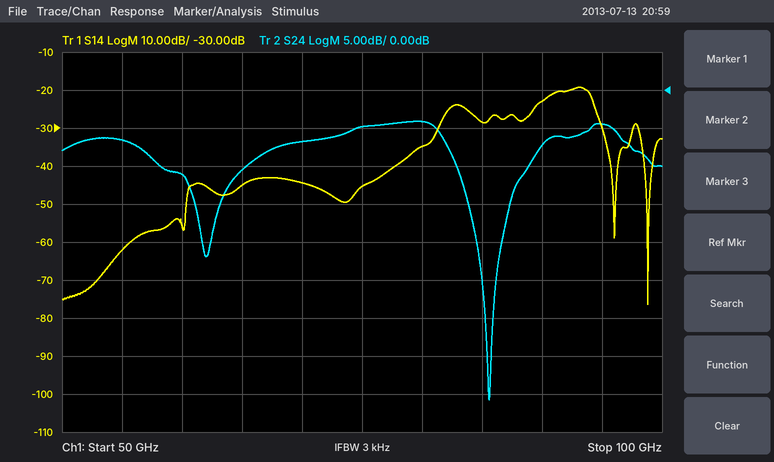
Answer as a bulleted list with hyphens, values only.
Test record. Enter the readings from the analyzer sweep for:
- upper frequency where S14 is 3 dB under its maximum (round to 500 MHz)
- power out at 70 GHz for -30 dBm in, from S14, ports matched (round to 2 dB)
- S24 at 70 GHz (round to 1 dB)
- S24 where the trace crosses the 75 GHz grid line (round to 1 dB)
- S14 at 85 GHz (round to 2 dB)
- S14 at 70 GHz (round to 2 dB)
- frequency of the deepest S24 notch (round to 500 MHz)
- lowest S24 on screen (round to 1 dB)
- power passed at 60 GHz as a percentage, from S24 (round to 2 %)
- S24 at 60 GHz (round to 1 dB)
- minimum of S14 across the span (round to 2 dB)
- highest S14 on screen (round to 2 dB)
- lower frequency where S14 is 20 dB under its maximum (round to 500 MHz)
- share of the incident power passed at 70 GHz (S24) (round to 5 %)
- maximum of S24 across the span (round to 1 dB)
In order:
- 94.0 GHz
- -74 dBm
- -7 dB
- -5 dB
- -28 dB
- -44 dB
- 85.5 GHz
- -41 dB
- 8 %
- -11 dB
- -76 dB
- -20 dB
- 78.0 GHz
- 20 %
- -4 dB
